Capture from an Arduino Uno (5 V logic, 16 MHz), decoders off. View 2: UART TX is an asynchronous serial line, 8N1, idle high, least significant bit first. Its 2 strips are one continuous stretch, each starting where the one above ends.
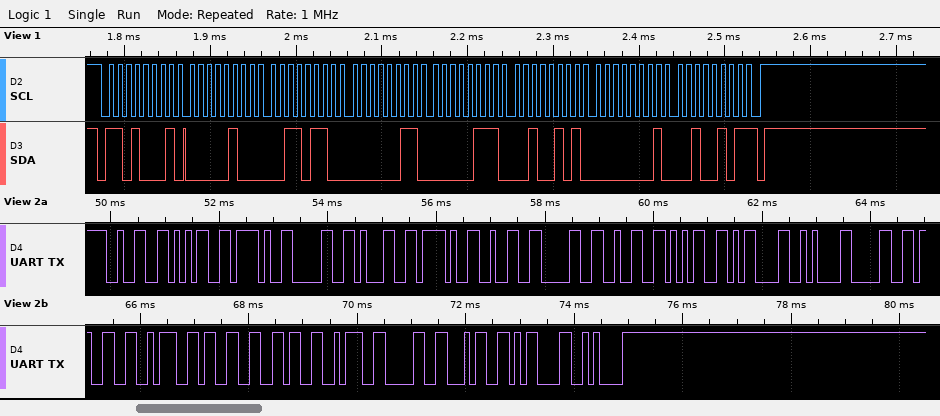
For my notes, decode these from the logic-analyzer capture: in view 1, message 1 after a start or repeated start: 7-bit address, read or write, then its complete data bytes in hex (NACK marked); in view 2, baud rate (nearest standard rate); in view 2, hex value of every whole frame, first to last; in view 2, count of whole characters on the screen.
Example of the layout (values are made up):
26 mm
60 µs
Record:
0x68 read: 04 36 03 07 25 01 25 NACK
9600 baud
32 35 2F 30 31 2F 32 30 32 35 0D 0A 30 33 3A 33 36 3A 30 34 0D 0A
22
